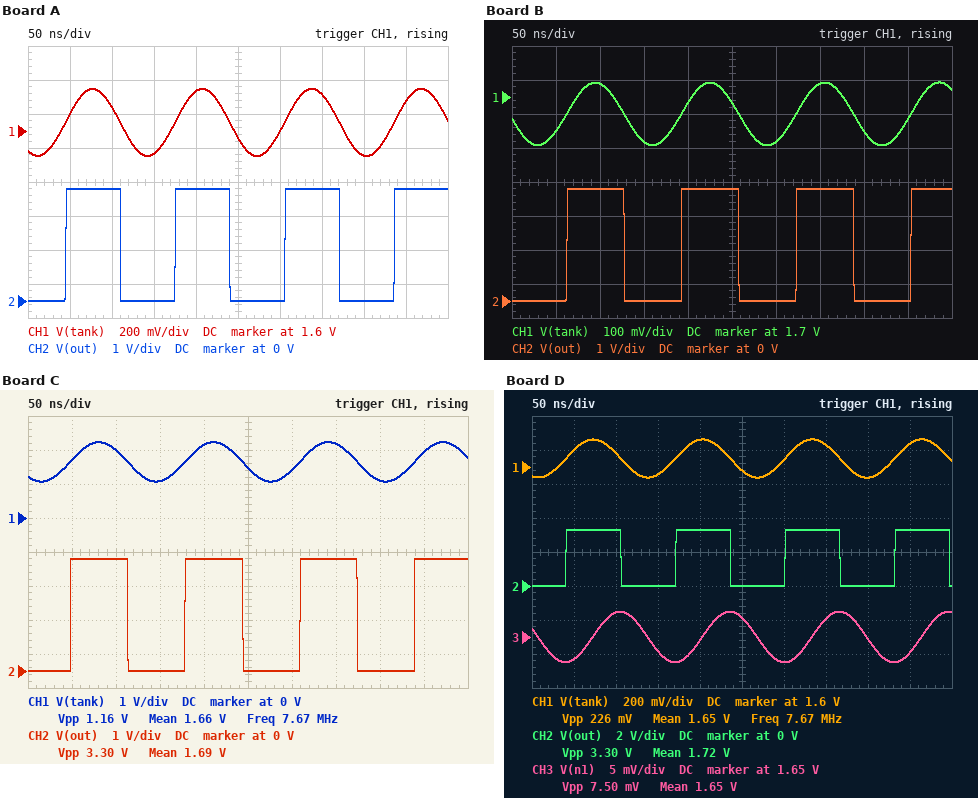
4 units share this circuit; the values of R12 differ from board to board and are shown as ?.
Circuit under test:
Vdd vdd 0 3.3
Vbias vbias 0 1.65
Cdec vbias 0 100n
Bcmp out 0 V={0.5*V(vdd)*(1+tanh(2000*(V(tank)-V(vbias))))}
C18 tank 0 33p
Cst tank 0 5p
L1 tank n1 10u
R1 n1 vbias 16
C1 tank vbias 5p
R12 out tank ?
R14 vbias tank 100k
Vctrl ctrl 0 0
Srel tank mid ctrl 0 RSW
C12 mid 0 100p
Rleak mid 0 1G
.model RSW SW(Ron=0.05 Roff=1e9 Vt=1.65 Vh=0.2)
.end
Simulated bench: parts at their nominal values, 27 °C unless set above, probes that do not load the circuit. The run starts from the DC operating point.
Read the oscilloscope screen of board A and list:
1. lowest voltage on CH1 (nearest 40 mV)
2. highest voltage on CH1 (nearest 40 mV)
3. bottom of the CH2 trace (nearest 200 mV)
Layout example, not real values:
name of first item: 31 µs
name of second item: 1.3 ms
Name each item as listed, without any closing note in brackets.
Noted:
lowest voltage on CH1: 1.44 V
highest voltage on CH1: 1.84 V
bottom of the CH2 trace: 0 V
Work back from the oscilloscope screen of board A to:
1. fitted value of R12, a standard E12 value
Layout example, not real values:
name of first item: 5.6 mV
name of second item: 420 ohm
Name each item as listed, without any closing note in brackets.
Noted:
fitted value of R12, a standard E12 value: 120 kΩ
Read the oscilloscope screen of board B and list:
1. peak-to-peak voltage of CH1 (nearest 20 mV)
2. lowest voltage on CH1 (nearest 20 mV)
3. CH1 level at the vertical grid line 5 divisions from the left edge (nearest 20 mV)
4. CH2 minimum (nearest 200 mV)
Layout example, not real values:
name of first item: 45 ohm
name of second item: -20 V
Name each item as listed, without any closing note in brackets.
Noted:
peak-to-peak voltage of CH1: 180 mV
lowest voltage on CH1: 1.56 V
CH1 level at the vertical grid line 5 divisions from the left edge: 1.68 V
CH2 minimum: 0 V
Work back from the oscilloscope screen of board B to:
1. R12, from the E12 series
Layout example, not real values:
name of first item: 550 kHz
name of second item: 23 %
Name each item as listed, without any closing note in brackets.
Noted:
R12, from the E12 series: 270 kΩ
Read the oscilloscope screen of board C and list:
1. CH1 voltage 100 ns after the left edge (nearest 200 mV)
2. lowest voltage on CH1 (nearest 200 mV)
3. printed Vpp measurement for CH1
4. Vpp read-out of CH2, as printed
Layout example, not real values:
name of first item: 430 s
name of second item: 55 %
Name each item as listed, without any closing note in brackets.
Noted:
CH1 voltage 100 ns after the left edge: 2.0 V
lowest voltage on CH1: 1.0 V
printed Vpp measurement for CH1: 1.16 V
Vpp read-out of CH2, as printed: 3.30 V
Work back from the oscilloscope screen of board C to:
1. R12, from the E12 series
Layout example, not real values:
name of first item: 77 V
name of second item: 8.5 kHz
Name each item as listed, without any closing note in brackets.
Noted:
R12, from the E12 series: 33 kΩ
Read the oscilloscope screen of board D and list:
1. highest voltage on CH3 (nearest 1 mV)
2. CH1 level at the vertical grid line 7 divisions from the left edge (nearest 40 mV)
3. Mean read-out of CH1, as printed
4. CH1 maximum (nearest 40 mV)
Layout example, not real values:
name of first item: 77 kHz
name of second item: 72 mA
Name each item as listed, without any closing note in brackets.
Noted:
highest voltage on CH3: 1.654 V
CH1 level at the vertical grid line 7 divisions from the left edge: 1.72 V
Mean read-out of CH1, as printed: 1.65 V
CH1 maximum: 1.76 V
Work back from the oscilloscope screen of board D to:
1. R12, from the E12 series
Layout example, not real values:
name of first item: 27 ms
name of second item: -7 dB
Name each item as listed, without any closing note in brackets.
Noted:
R12, from the E12 series: 220 kΩ
